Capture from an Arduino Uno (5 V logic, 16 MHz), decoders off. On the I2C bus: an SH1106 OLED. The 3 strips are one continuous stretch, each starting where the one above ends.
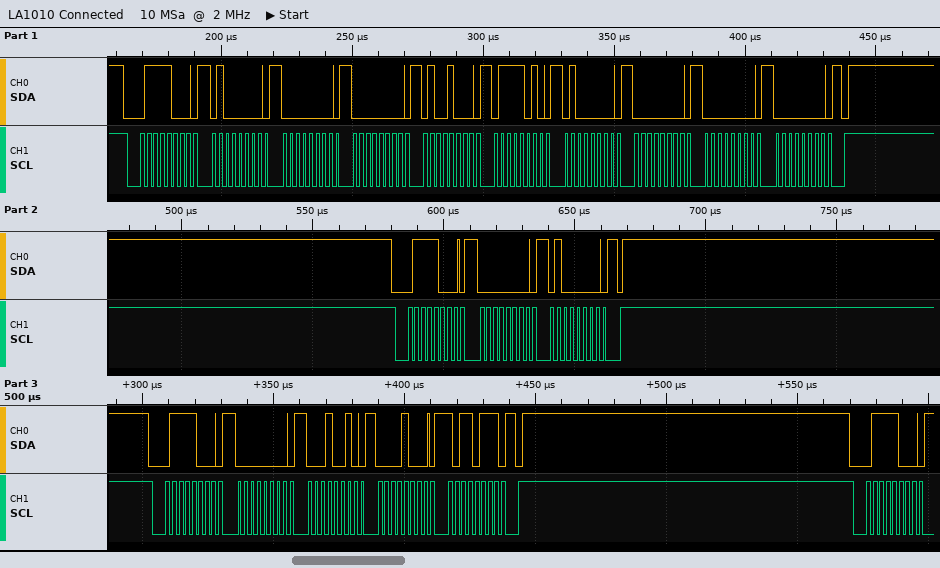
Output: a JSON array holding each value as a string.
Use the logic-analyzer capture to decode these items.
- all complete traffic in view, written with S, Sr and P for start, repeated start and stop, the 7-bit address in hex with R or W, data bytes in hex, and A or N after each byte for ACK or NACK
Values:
["S 3CW A 40 A 00 A 00 A 48 A 7A A 40 A 00 A 00 A 00 A P S 3CW A 00 A 40 A P S 3CW A 00 A 12 A 08 A B7 A P S 3CW A"]
